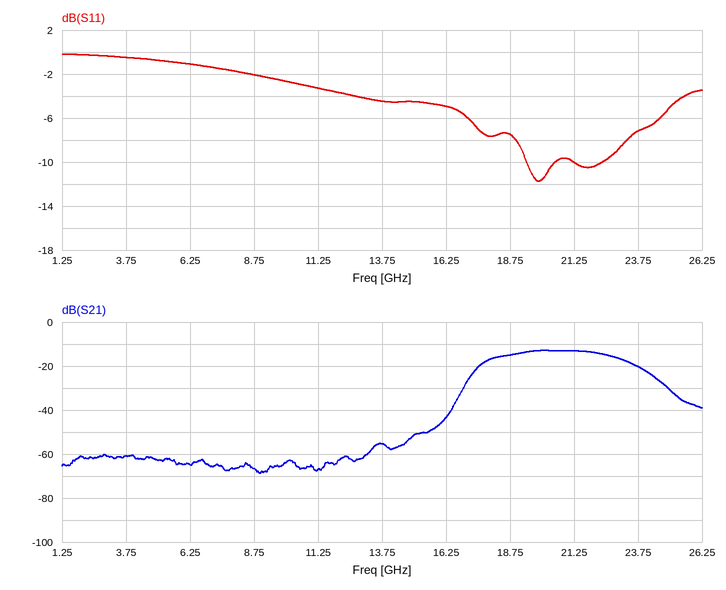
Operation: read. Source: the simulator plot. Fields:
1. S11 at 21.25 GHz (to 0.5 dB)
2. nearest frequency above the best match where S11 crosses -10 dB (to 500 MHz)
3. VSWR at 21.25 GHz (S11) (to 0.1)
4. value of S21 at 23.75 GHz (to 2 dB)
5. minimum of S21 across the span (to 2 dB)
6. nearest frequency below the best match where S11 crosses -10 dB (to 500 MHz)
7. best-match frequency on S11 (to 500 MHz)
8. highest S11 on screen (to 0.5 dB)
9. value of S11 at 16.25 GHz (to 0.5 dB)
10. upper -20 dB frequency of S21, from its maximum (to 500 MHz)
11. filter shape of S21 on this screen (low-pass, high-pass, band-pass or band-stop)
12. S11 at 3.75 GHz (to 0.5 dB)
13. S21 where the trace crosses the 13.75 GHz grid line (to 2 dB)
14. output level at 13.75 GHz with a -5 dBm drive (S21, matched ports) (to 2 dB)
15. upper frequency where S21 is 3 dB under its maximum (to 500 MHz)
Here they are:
-10.0 dB
20.5 GHz
1.9
-20 dB
-68 dB
19.5 GHz
20.0 GHz
0.0 dB
-5.0 dB
25.0 GHz
band-pass
-0.5 dB
-56 dB
-60 dBm
23.0 GHz
